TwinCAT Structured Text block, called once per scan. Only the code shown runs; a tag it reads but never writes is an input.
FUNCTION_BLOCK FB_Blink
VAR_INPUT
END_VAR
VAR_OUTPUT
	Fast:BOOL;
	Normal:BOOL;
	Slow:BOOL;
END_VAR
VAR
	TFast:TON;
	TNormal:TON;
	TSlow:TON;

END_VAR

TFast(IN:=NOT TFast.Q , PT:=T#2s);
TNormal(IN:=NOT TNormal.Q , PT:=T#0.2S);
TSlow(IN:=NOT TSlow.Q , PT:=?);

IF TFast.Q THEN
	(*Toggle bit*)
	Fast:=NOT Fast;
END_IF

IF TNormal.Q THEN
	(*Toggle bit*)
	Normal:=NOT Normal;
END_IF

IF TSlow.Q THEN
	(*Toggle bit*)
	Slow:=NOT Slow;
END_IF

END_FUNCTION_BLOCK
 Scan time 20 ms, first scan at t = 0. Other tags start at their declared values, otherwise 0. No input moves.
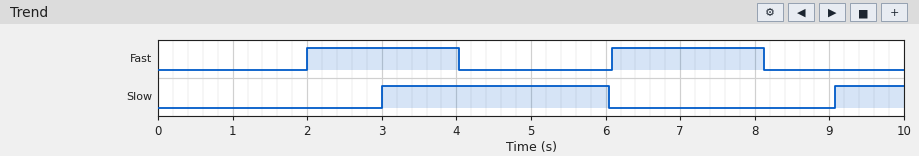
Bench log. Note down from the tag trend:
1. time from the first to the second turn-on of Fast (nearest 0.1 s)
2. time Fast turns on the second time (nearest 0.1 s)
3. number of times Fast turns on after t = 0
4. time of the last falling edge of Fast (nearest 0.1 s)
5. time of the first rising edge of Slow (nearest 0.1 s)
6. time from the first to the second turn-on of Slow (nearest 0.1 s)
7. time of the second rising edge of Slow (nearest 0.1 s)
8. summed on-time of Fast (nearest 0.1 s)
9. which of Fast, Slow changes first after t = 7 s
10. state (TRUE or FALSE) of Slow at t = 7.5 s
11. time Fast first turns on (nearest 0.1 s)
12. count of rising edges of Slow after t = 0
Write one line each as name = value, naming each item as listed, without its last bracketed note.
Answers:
time from the first to the second turn-on of Fast = 4.1 s
time Fast turns on the second time = 6.1 s
number of times Fast turns on after t = 0 = 2
time of the last falling edge of Fast = 8.1 s
time of the first rising edge of Slow = 3.0 s
time from the first to the second turn-on of Slow = 6.1 s
time of the second rising edge of Slow = 9.1 s
summed on-time of Fast = 4.1 s
which of Fast, Slow changes first after t = 7 s = Fast
state (TRUE or FALSE) of Slow at t = 7.5 s = FALSE
time Fast first turns on = 2.0 s
count of rising edges of Slow after t = 0 = 2
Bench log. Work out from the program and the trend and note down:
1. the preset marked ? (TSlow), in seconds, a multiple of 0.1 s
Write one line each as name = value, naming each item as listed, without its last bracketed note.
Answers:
the preset marked ? (TSlow), in seconds, a multiple of 0.1 s = 3.0 s
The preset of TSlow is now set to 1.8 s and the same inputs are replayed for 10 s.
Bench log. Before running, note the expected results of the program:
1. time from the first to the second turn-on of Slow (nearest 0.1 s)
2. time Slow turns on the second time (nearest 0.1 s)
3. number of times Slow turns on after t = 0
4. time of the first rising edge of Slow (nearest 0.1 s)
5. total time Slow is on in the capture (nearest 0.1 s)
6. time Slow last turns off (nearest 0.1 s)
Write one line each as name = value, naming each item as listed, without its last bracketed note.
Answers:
time from the first to the second turn-on of Slow = 3.7 s
time Slow turns on the second time = 5.5 s
number of times Slow turns on after t = 0 = 3
time of the first rising edge of Slow = 1.8 s
total time Slow is on in the capture = 4.5 s
time Slow last turns off = 7.3 s
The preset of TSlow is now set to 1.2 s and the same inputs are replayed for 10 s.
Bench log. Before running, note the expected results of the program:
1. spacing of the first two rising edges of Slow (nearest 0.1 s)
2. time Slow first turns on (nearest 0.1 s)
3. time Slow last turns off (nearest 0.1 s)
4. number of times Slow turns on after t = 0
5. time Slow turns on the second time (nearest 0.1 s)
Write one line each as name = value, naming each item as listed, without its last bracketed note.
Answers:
spacing of the first two rising edges of Slow = 2.5 s
time Slow first turns on = 1.2 s
time Slow last turns off = 9.9 s
number of times Slow turns on after t = 0 = 4
time Slow turns on the second time = 3.7 s
